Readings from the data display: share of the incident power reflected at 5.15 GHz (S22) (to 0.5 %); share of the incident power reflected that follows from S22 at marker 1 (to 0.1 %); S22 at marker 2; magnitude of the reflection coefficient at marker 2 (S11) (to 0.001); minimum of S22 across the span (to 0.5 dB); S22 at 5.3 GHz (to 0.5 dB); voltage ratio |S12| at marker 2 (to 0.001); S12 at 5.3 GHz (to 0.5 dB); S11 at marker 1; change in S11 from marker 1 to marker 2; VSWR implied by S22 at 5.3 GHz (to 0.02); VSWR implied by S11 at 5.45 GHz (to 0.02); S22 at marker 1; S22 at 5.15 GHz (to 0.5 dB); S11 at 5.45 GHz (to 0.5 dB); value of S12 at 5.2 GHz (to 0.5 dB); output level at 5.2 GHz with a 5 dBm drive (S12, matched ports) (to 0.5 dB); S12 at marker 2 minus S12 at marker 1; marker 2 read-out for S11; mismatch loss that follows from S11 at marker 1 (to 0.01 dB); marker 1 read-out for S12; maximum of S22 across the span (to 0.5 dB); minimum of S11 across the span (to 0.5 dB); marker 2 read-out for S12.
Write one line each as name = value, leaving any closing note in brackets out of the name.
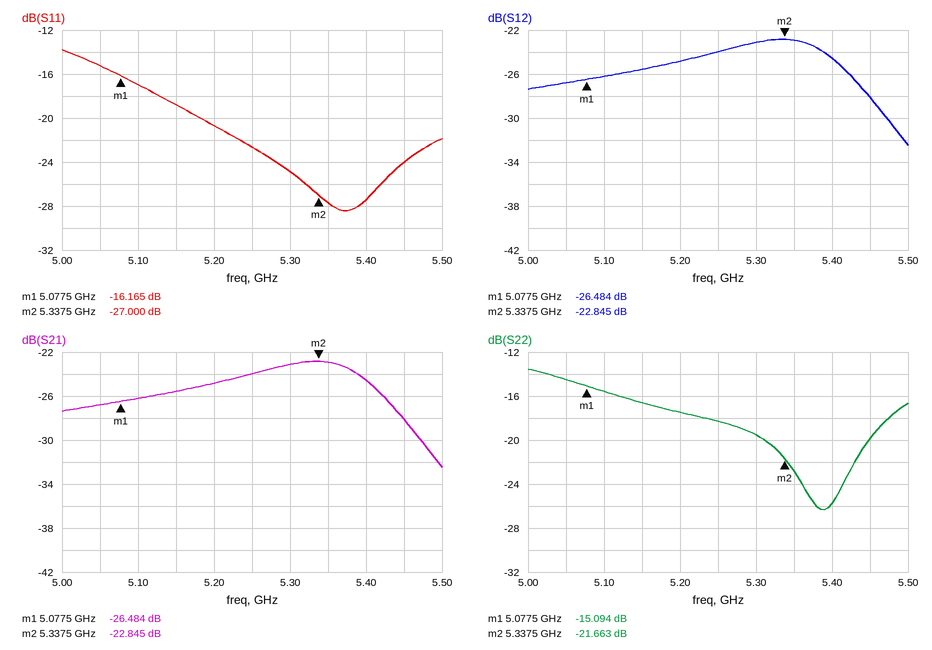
share of the incident power reflected at 5.15 GHz (S22) = 2.0 %
share of the incident power reflected that follows from S22 at marker 1 = 3.1 %
S22 at marker 2 = -21.663 dB
magnitude of the reflection coefficient at marker 2 (S11) = 0.045
minimum of S22 across the span = -26.5 dB
S22 at 5.3 GHz = -19.5 dB
voltage ratio |S12| at marker 2 = 0.072
S12 at 5.3 GHz = -23.0 dB
S11 at marker 1 = -16.165 dB
change in S11 from marker 1 to marker 2 = -10.835 dB
VSWR implied by S22 at 5.3 GHz = 1.24
VSWR implied by S11 at 5.45 GHz = 1.14
S22 at marker 1 = -15.094 dB
S22 at 5.15 GHz = -16.5 dB
S11 at 5.45 GHz = -24.0 dB
value of S12 at 5.2 GHz = -25.0 dB
output level at 5.2 GHz with a 5 dBm drive (S12, matched ports) = -20.0 dBm
S12 at marker 2 minus S12 at marker 1 = 3.639 dB
marker 2 read-out for S11 = -27.000 dB
mismatch loss that follows from S11 at marker 1 = 0.11 dB
marker 1 read-out for S12 = -26.484 dB
maximum of S22 across the span = -13.5 dB
minimum of S11 across the span = -28.5 dB
marker 2 read-out for S12 = -22.845 dB
